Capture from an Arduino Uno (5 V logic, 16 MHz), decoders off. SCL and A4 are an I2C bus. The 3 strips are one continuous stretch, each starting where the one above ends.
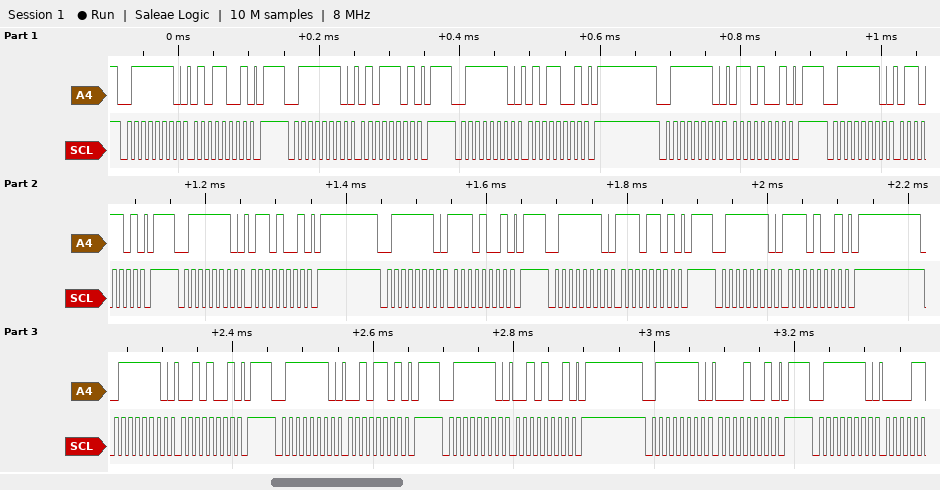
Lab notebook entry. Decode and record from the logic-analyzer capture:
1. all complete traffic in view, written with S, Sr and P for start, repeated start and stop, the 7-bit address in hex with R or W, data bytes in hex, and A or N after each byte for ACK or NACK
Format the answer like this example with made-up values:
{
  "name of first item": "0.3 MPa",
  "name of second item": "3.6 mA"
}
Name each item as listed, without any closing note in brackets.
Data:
{
  "all complete traffic in view, written with S, Sr and P for start, repeated start and stop, the 7-bit address in hex with R or W, data bytes in hex, and A or N after each byte for ACK or NACK": "S 3FW A 59 A P S 3FW A 5D A P S 3FW A 59 A P S 3FW A 69 A P S 3FW A 6D A P S 3FW A 69 A P S 3FW A E9 A P S 3FW A ED A P S 3FW A E9 A P S 3FW A 29 A P S 3FW A 2D A P S 3FW A 29 A P S 3FW A 09 A P S 3FW A"
}
